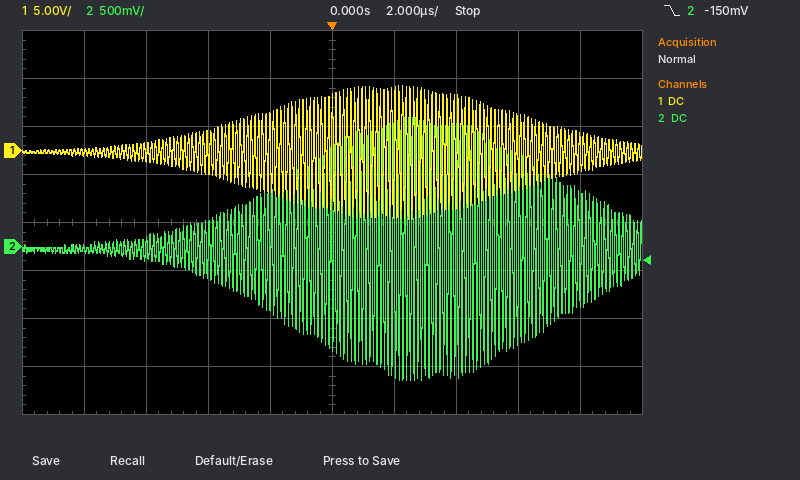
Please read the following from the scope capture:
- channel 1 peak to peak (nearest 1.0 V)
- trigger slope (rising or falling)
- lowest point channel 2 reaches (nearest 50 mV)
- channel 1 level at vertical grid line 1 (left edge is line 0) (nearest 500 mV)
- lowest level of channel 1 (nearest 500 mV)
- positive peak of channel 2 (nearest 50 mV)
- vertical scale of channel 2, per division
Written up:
14.0 V
falling
-1.40 V
0.0 V
-7.0 V
1.35 V
500 mV
